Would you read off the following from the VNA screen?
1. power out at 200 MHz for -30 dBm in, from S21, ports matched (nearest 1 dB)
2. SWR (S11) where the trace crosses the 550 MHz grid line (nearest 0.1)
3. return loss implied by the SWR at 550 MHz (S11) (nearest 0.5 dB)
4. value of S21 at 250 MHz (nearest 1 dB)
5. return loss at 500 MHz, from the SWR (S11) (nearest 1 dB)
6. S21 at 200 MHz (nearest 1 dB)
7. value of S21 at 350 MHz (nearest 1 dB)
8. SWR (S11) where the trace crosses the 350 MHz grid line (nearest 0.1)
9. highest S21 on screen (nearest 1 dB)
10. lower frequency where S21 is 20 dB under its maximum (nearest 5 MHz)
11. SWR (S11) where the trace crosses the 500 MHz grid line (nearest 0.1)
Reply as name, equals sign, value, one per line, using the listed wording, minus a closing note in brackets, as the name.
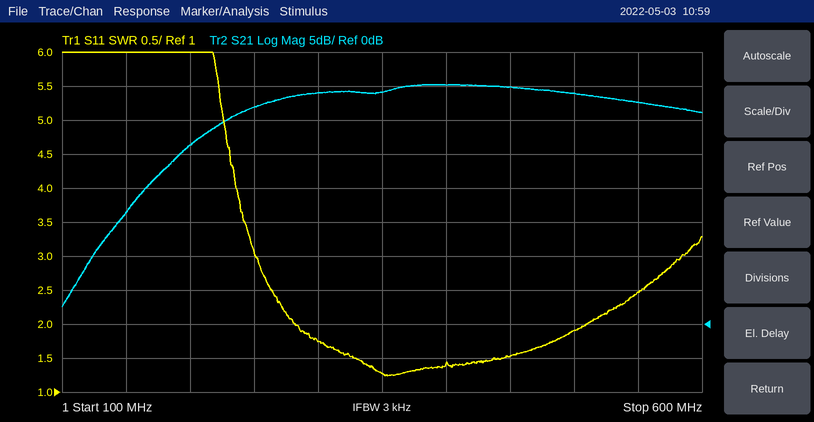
power out at 200 MHz for -30 dBm in, from S21, ports matched = -4 dBm
SWR (S11) where the trace crosses the 550 MHz grid line = 2.5
return loss implied by the SWR at 550 MHz (S11) = 7.5 dB
value of S21 at 250 MHz = 32 dB
return loss at 500 MHz, from the SWR (S11) = 10 dB
S21 at 200 MHz = 26 dB
value of S21 at 350 MHz = 34 dB
SWR (S11) where the trace crosses the 350 MHz grid line = 1.3
highest S21 on screen = 35 dB
lower frequency where S21 is 20 dB under its maximum = 145 MHz
SWR (S11) where the trace crosses the 500 MHz grid line = 1.9
